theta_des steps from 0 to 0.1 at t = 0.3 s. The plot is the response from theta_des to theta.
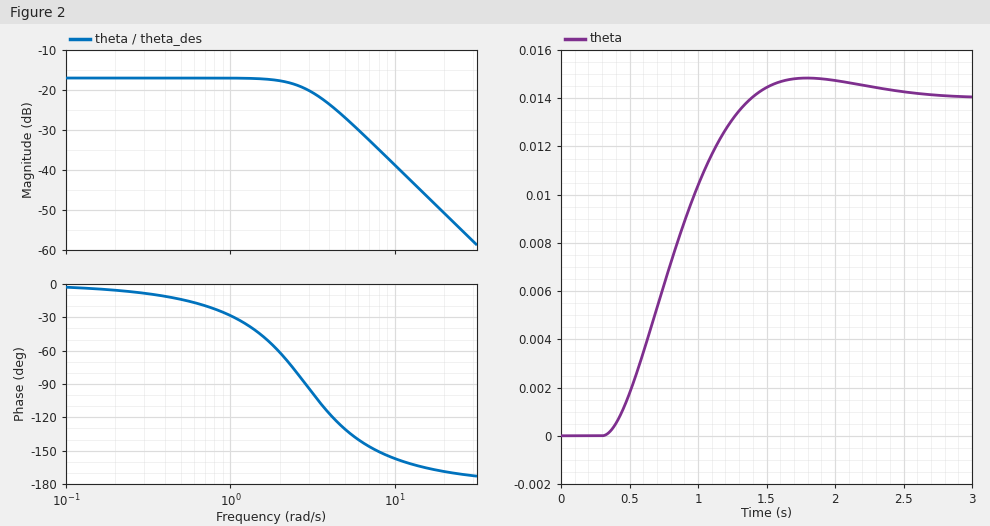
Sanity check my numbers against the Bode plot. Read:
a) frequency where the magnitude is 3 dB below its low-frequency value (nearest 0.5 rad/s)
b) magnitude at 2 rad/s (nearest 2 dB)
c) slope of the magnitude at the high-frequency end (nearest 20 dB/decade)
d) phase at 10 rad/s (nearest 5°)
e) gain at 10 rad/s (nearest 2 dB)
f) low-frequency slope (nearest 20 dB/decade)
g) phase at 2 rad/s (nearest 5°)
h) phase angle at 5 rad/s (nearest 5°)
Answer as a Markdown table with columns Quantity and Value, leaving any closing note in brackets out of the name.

| Quantity | Value |
|---|---|
| frequency where the magnitude is 3 dB below its low-frequency value | 3.0 rad/s |
| magnitude at 2 rad/s | -18 dB |
| slope of the magnitude at the high-frequency end | -40 dB/decade |
| phase at 10 rad/s | -155° |
| gain at 10 rad/s | -38 dB |
| low-frequency slope | 0 dB/decade |
| phase at 2 rad/s | -60° |
| phase angle at 5 rad/s | -130° |
